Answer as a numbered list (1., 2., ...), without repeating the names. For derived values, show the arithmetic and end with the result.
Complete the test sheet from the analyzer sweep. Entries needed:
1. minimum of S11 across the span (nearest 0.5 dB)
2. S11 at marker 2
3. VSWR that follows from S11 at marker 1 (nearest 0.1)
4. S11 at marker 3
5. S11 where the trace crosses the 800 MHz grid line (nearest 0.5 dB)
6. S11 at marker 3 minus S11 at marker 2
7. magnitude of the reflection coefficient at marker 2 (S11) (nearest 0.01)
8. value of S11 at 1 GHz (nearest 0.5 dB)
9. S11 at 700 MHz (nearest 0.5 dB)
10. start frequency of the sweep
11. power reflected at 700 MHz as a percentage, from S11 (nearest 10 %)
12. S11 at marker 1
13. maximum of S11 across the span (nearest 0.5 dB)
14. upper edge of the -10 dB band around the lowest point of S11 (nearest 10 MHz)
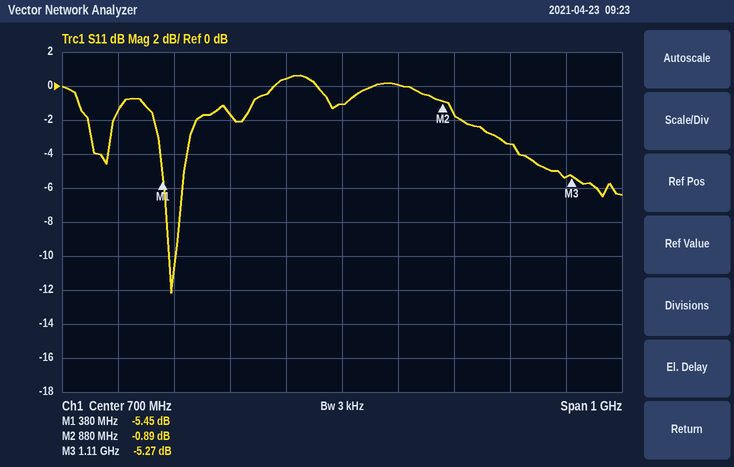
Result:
1. -12.0 dB
2. -0.89 dB
3. (1 + 0.5339)/(1 − 0.5339) ≈ 3.3
4. -5.27 dB
5. 0.0 dB
6. -5.27 − (-0.89) = -4.38 dB
7. 10^(-0.89/20) ≈ 0.90
8. -3.5 dB
9. -1.0 dB
10. 200 MHz
11. 10^(-1/10) ≈ 79.4 %, so 80 % to the nearest 10 %
12. -5.45 dB
13. 0.5 dB
14. 400 MHz
